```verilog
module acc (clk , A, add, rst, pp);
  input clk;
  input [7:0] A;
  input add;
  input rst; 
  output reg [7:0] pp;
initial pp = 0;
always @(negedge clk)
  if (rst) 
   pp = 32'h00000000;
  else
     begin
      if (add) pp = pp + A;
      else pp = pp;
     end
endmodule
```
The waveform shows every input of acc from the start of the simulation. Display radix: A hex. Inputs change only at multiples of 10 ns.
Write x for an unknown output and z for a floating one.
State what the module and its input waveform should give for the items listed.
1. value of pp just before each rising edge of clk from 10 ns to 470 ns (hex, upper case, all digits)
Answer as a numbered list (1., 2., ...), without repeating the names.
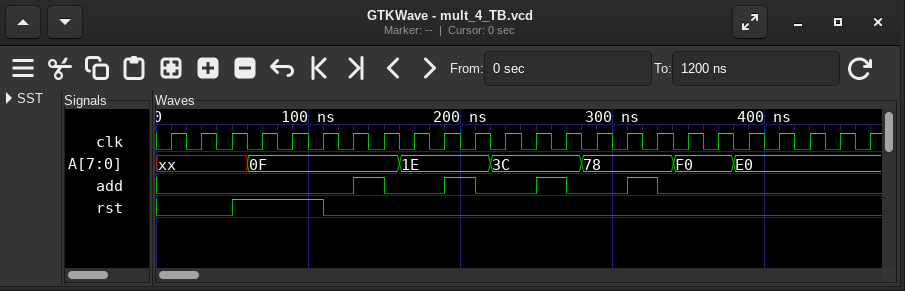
1. 00, 00, 00, 00, 00, 00, 00, 0F, 0F, 0F, 2D, 2D, 2D, 69, 69, 69, E1, E1, E1, E1, E1, E1, E1, E1
